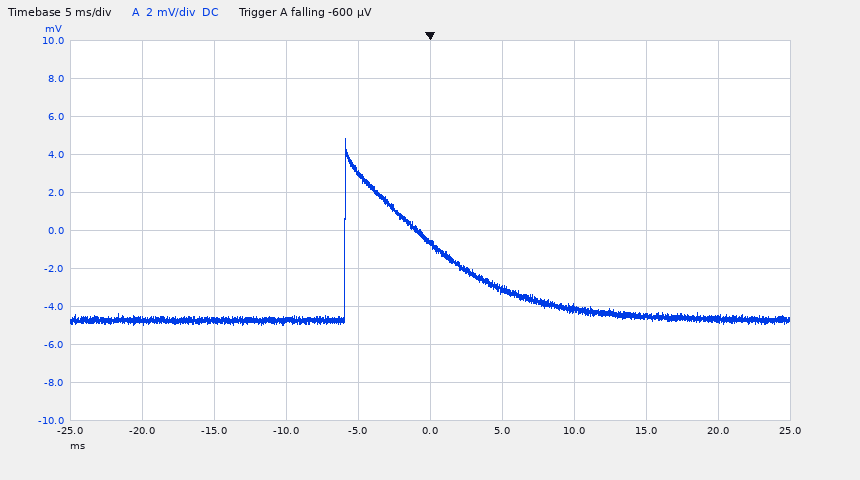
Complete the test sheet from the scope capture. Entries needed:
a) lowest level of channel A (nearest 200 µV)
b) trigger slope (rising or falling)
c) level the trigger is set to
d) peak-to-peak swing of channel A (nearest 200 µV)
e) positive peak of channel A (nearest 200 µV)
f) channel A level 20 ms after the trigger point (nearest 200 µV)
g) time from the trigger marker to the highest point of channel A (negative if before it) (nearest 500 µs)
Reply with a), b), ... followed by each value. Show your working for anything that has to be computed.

a) -5.0 mV
b) falling
c) -600 µV
d) 4.8 mV − (-5.0 mV) = 9.8 mV
e) 4.8 mV
f) -4.6 mV
g) -6.0 ms
